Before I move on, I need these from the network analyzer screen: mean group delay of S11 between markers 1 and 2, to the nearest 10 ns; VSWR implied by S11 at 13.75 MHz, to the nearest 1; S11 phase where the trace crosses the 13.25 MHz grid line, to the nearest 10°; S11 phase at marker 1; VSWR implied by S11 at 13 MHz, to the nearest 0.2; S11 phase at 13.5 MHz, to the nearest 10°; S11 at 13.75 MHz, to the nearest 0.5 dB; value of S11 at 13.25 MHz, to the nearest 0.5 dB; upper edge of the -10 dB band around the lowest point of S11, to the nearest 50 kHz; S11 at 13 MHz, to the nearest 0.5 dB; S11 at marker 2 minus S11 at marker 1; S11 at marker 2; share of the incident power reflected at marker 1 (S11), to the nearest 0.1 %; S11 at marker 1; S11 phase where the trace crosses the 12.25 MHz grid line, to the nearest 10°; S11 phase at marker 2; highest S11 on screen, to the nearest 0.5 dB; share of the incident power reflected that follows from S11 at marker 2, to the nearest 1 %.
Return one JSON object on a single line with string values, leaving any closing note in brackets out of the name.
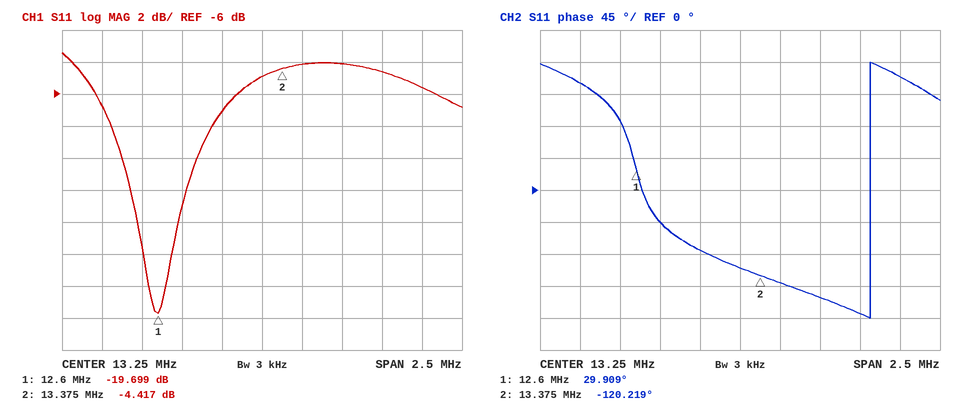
{"mean group delay of S11 between markers 1 and 2, to the nearest 10 ns": "540 ns", "VSWR implied by S11 at 13.75 MHz, to the nearest 1": "4", "S11 phase where the trace crosses the 13.25 MHz grid line, to the nearest 10°": "-110°", "S11 phase at marker 1": "29.909°", "VSWR implied by S11 at 13 MHz, to the nearest 0.2": "2.6", "S11 phase at 13.5 MHz, to the nearest 10°": "-130°", "S11 at 13.75 MHz, to the nearest 0.5 dB": "-4.0 dB", "value of S11 at 13.25 MHz, to the nearest 0.5 dB": "-5.0 dB", "upper edge of the -10 dB band around the lowest point of S11, to the nearest 50 kHz": "12.85 MHz", "S11 at 13 MHz, to the nearest 0.5 dB": "-7.0 dB", "S11 at marker 2 minus S11 at marker 1": "15.282 dB", "S11 at marker 2": "-4.417 dB", "share of the incident power reflected at marker 1 (S11), to the nearest 0.1 %": "1.1 %", "S11 at marker 1": "-19.699 dB", "S11 phase where the trace crosses the 12.25 MHz grid line, to the nearest 10°": "150°", "S11 phase at marker 2": "-120.219°", "highest S11 on screen, to the nearest 0.5 dB": "-3.5 dB", "share of the incident power reflected that follows from S11 at marker 2, to the nearest 1 %": "36 %"}
